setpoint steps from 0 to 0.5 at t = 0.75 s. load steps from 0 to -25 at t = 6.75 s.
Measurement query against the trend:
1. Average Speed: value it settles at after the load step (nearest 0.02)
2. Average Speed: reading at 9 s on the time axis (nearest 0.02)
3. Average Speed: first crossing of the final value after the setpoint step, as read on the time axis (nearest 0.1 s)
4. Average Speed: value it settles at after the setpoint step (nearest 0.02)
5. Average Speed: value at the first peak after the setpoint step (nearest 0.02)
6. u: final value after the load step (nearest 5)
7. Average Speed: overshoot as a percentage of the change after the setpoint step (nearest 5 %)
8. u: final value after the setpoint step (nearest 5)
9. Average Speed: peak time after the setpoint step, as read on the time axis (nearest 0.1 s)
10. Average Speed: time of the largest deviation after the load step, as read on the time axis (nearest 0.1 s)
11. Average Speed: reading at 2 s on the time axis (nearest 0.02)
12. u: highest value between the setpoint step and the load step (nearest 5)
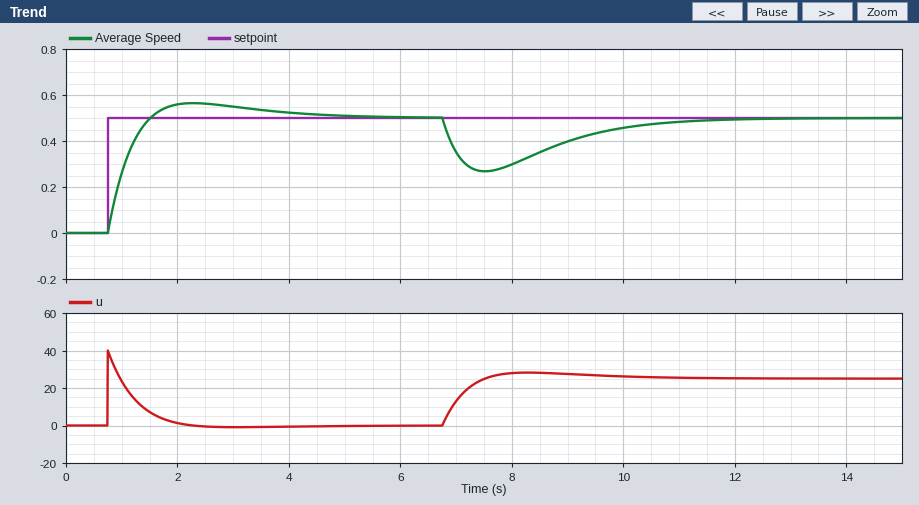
0.50
0.40
1.5 s
0.50
0.56
25
15 %
0
2.3 s
7.5 s
0.56
40
